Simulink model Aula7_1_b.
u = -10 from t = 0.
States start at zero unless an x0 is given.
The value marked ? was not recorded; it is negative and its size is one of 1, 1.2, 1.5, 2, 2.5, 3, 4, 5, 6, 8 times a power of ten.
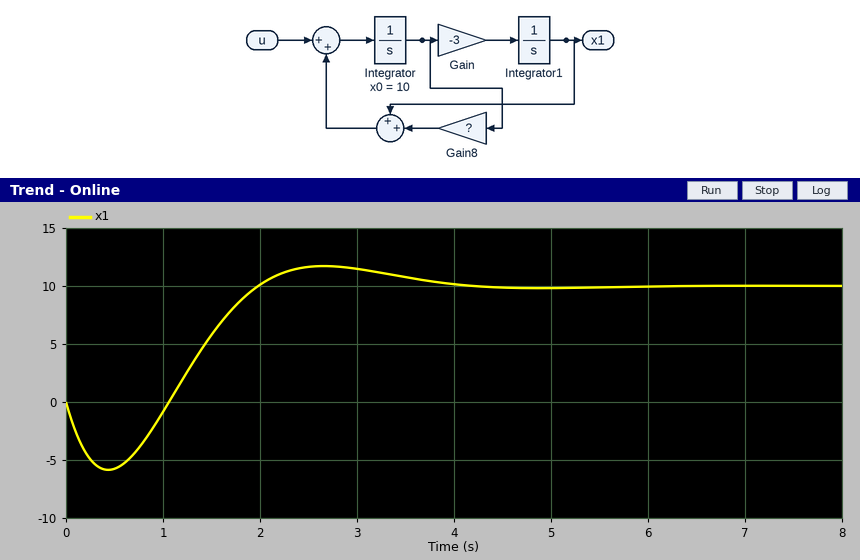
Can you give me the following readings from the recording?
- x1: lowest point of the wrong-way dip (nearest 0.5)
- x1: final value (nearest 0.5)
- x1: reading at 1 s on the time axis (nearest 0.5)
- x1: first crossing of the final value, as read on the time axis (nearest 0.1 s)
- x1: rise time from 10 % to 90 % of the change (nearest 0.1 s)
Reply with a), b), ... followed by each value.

a) -6.0
b) 10.0
c) -1.0
d) 2.0 s
e) 0.7 s
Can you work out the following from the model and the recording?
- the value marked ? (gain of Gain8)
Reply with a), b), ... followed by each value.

a) -2
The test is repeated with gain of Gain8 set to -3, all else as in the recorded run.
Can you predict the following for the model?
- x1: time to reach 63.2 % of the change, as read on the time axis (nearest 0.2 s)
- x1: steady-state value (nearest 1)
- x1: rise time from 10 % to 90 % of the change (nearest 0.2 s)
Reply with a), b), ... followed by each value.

a) 1.8 s
b) 10
c) 1.4 s
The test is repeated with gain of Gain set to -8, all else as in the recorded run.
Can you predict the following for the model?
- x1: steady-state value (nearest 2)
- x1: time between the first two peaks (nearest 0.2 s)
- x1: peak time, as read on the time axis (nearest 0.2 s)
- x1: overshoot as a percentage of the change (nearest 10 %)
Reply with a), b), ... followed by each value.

a) 10
b) 2.4 s
c) 1.6 s
d) 70 %
